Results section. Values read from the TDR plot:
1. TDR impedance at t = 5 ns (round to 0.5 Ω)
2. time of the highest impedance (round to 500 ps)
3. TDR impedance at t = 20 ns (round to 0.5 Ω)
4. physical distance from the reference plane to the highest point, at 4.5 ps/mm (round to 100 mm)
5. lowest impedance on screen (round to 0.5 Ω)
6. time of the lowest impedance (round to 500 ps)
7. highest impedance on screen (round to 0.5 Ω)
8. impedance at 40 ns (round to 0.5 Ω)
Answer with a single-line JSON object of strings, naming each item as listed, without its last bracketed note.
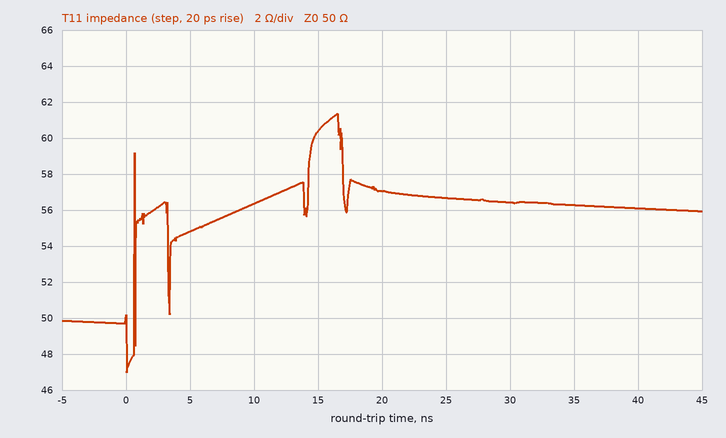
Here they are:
{"TDR impedance at t = 5 ns": "55.0 Ω", "time of the highest impedance": "16.5 ns", "TDR impedance at t = 20 ns": "57.0 Ω", "physical distance from the reference plane to the highest point, at 4.5 ps/mm": "1.8 m", "lowest impedance on screen": "47.0 Ω", "time of the lowest impedance": "0.0 ns", "highest impedance on screen": "61.5 Ω", "impedance at 40 ns": "56.0 Ω"}
